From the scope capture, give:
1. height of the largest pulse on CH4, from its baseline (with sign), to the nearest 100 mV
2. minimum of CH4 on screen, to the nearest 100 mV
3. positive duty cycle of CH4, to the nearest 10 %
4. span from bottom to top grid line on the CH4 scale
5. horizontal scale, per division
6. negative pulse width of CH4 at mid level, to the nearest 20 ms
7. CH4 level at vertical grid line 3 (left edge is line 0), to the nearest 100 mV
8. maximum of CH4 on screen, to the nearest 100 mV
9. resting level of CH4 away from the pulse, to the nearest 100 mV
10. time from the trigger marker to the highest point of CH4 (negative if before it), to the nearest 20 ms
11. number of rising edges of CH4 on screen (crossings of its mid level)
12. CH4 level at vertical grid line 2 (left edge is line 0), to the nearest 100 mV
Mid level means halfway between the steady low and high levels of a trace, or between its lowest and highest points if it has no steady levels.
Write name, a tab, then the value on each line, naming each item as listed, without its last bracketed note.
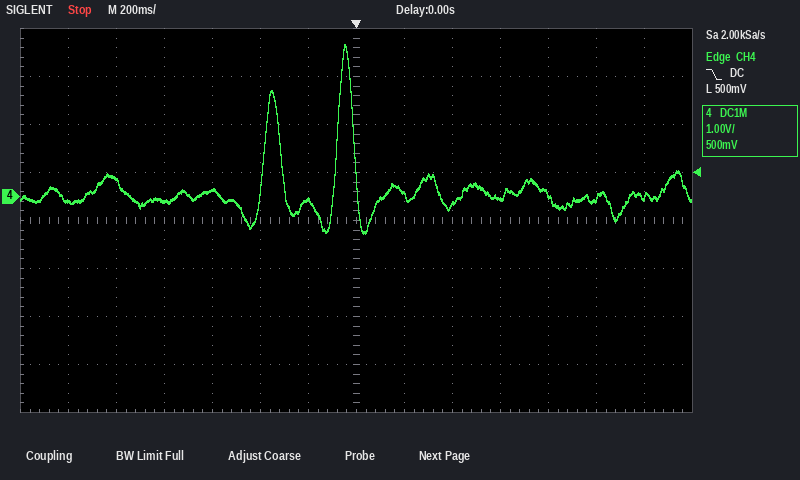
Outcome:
height of the largest pulse on CH4, from its baseline (with sign), to the nearest 100 mV	+3.2 V
minimum of CH4 on screen, to the nearest 100 mV	-800 mV
positive duty cycle of CH4, to the nearest 10 %	20 %
span from bottom to top grid line on the CH4 scale	8 V
horizontal scale, per division	200 ms
negative pulse width of CH4 at mid level, to the nearest 20 ms	240 ms
CH4 level at vertical grid line 3 (left edge is line 0), to the nearest 100 mV	-100 mV
maximum of CH4 on screen, to the nearest 100 mV	3.2 V
resting level of CH4 away from the pulse, to the nearest 100 mV	0.0 V
time from the trigger marker to the highest point of CH4 (negative if before it), to the nearest 20 ms	-40 ms
number of rising edges of CH4 on screen	2
CH4 level at vertical grid line 2 (left edge is line 0), to the nearest 100 mV	400 mV
